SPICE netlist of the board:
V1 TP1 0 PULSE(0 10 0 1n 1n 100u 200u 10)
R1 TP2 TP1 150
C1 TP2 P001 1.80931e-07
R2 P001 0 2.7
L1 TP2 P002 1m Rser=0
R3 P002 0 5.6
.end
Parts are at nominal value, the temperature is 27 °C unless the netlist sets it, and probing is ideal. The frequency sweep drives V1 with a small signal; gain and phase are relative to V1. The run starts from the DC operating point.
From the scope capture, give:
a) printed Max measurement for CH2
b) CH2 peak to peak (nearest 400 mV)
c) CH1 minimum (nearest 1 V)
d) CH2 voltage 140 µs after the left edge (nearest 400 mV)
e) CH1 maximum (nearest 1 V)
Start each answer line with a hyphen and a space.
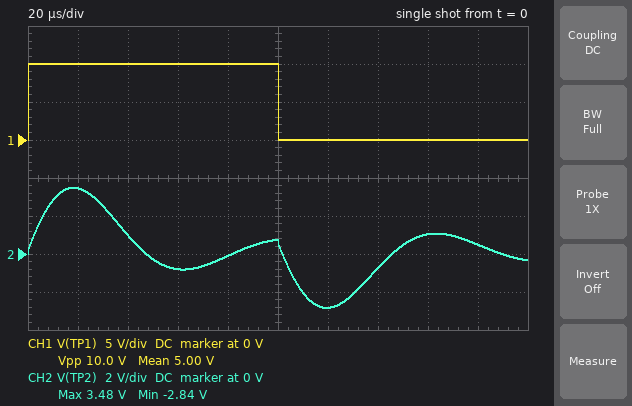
- 3.48 V
- 6.4 V
- 0 V
- -800 mV
- 10 V
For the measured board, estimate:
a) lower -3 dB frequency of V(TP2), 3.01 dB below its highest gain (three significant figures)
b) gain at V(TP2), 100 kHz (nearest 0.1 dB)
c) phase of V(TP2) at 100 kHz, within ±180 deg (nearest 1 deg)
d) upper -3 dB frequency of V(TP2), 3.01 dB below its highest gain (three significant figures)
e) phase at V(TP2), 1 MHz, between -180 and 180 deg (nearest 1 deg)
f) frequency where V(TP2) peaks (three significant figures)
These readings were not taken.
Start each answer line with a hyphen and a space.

- 8.91 kHz
- -24.3 dB
- -69 deg
- 16.0 kHz
- -18 deg
- 11.9 kHz
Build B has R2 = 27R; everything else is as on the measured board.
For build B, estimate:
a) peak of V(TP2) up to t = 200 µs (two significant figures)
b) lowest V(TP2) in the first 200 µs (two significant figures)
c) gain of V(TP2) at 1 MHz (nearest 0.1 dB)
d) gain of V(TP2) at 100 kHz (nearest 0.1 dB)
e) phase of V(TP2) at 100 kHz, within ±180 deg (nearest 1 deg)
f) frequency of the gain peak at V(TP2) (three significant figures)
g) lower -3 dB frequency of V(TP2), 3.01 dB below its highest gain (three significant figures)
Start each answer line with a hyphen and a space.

- 3.0 V
- -2.5 V
- -16.3 dB
- -15.8 dB
- -13 deg
- 11.3 kHz
- 7.47 kHz
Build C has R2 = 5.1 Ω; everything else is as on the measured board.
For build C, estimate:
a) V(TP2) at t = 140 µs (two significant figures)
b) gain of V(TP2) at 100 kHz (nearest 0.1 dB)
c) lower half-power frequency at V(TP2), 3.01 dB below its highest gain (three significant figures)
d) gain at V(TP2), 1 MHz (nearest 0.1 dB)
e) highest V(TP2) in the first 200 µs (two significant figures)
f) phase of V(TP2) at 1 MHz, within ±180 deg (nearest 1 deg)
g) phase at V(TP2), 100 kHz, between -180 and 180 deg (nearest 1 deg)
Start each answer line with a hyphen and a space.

- -690 mV
- -23.6 dB
- 8.73 kHz
- -29.5 dB
- 3.4 V
- -9 deg
- -56 deg
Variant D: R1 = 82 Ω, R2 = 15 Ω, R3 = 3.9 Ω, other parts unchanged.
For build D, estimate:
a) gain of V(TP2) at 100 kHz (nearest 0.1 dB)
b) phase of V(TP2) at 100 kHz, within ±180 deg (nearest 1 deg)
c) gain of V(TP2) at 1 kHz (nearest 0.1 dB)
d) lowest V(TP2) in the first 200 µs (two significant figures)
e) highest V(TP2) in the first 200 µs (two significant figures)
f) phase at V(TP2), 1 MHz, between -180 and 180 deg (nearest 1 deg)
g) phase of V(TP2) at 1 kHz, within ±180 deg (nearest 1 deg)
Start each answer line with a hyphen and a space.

- -14.9 dB
- -24 deg
- -21.3 dB
- -4.1 V
- 4.6 V
- -3 deg
- 54 deg
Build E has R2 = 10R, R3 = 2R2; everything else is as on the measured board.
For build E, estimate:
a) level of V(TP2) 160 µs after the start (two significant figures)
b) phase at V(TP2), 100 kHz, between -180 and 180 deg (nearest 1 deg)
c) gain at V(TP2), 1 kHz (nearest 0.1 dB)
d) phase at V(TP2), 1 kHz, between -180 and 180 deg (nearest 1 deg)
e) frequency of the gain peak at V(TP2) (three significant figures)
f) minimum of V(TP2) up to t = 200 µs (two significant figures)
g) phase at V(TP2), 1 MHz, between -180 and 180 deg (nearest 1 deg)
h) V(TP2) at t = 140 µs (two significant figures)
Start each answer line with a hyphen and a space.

- 950 mV
- -37 deg
- -27.1 dB
- 68 deg
- 11.6 kHz
- -2.8 V
- -5 deg
- -610 mV
